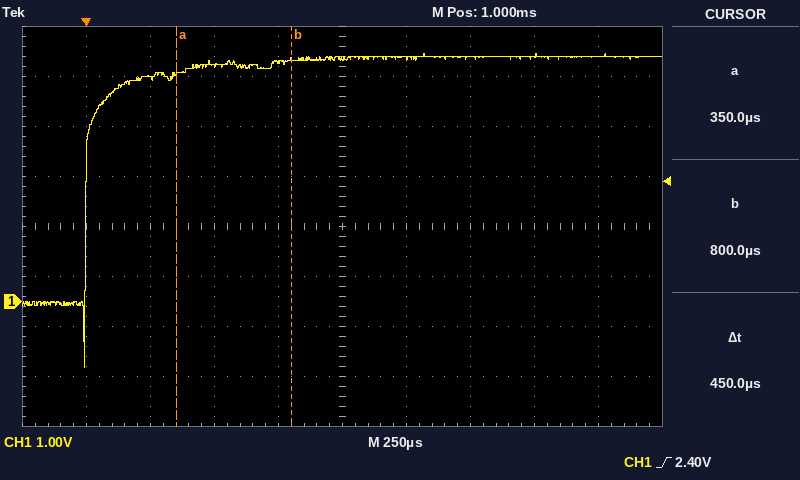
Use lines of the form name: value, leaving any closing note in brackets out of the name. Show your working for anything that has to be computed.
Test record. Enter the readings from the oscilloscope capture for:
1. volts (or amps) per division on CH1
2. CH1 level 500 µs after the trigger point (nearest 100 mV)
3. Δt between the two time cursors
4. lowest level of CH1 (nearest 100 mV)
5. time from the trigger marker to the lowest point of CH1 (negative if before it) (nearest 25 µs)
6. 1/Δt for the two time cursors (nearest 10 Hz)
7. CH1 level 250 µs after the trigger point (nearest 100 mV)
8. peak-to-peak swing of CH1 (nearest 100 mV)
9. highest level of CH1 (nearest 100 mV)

volts (or amps) per division on CH1: 1 V
CH1 level 500 µs after the trigger point: 4.7 V
Δt between the two time cursors: 450 µs
lowest level of CH1: -1.3 V
time from the trigger marker to the lowest point of CH1 (negative if before it): 0 µs
1/Δt for the two time cursors: 1 / 450 µs ≈ 2.22 kHz
CH1 level 250 µs after the trigger point: 4.5 V
peak-to-peak swing of CH1: 5.0 V − (-1.3 V) = 6.3 V
highest level of CH1: 5.0 V
